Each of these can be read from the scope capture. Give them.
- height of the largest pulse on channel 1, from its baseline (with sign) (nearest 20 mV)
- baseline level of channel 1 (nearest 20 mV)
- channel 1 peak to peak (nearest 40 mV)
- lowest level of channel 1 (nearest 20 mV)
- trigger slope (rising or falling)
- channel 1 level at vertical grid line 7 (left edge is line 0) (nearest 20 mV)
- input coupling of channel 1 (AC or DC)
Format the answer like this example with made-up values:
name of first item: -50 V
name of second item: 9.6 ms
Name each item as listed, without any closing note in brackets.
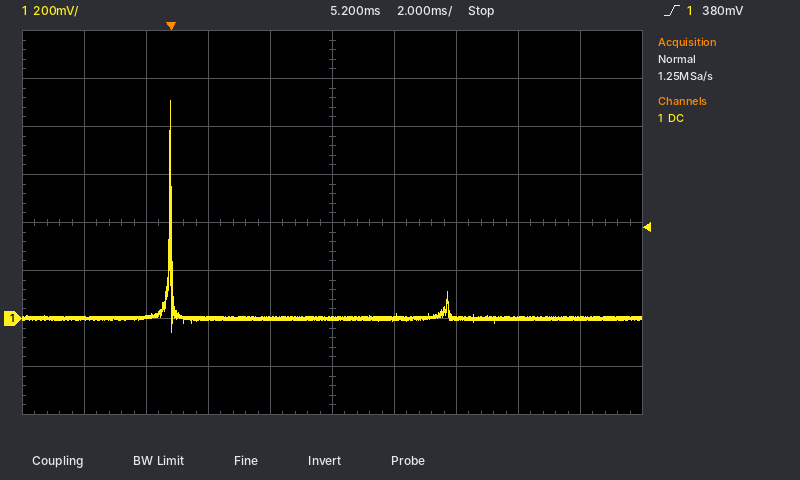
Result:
height of the largest pulse on channel 1, from its baseline (with sign): +900 mV
baseline level of channel 1: 0 mV
channel 1 peak to peak: 960 mV
lowest level of channel 1: -60 mV
trigger slope: rising
channel 1 level at vertical grid line 7 (left edge is line 0): 0 mV
input coupling of channel 1: DC
